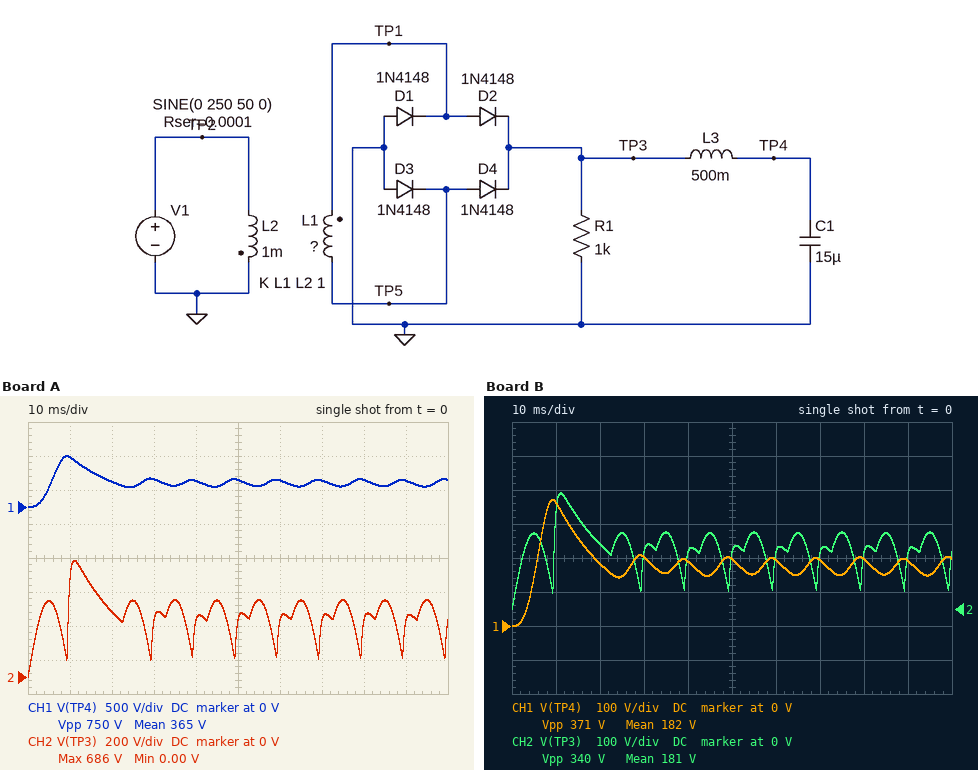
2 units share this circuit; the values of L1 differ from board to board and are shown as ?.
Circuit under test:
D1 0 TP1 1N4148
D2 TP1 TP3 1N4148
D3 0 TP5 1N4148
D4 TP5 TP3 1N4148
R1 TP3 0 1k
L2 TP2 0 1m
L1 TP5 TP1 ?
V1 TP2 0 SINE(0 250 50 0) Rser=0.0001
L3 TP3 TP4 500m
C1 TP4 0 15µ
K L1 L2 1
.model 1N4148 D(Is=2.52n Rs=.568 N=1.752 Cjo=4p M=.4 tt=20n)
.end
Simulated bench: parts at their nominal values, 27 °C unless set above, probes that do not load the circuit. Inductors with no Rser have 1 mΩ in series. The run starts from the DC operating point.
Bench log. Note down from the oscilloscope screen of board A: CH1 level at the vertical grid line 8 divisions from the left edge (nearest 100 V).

400 V
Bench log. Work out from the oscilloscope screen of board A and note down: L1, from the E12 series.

3.3 mH
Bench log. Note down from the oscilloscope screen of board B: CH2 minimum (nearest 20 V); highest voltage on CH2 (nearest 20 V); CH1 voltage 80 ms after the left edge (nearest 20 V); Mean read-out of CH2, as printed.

0 V
340 V
200 V
181 V
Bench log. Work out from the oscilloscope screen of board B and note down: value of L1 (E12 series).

820 µH
